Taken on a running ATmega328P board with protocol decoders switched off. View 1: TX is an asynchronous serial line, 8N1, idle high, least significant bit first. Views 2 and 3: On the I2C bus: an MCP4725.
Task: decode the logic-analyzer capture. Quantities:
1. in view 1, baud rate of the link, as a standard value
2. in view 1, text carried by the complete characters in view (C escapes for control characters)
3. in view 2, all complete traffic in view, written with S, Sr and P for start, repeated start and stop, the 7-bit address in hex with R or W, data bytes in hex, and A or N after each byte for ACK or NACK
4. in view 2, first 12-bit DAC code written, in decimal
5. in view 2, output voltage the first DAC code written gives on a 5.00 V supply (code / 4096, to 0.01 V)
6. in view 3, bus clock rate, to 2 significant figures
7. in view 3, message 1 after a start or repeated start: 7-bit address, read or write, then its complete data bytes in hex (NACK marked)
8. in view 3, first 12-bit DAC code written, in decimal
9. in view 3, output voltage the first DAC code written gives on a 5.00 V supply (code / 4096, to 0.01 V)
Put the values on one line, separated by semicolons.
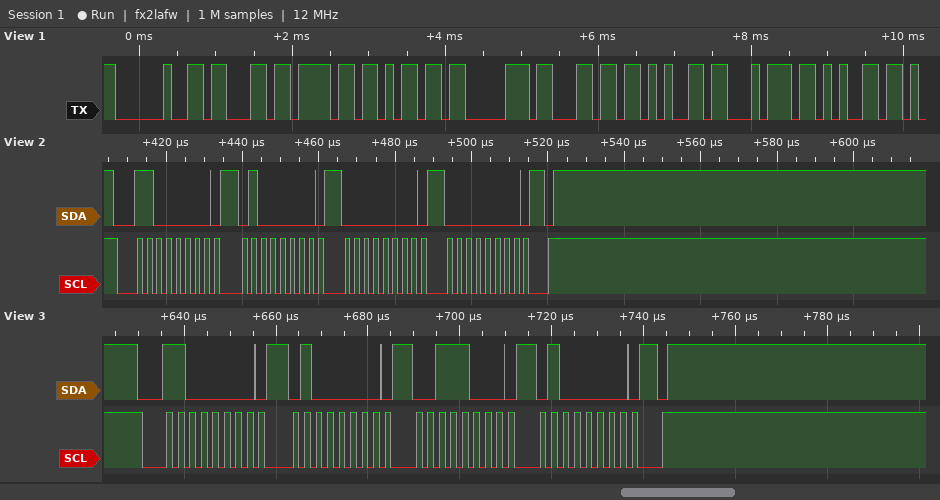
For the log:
9600 baud; " complete"; S 60W A 40 A 00 A 00 A P; 0; 0.00 V; 400 kHz; 0x60 write: 40 38 40; 900; 1.10 V
